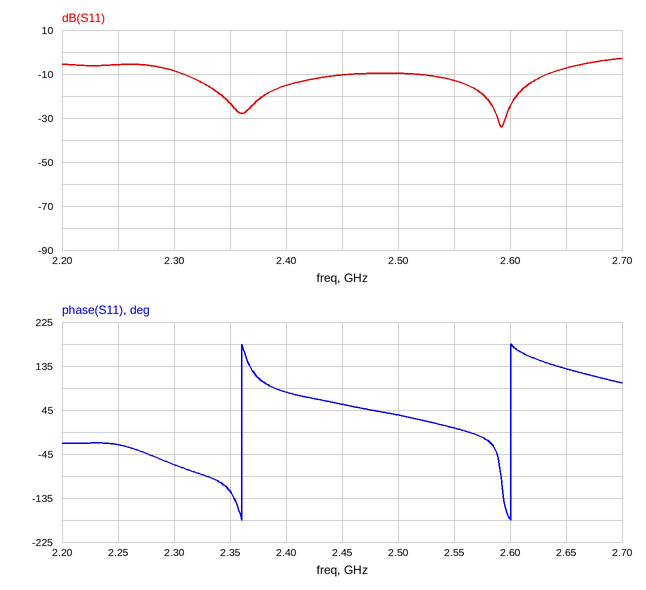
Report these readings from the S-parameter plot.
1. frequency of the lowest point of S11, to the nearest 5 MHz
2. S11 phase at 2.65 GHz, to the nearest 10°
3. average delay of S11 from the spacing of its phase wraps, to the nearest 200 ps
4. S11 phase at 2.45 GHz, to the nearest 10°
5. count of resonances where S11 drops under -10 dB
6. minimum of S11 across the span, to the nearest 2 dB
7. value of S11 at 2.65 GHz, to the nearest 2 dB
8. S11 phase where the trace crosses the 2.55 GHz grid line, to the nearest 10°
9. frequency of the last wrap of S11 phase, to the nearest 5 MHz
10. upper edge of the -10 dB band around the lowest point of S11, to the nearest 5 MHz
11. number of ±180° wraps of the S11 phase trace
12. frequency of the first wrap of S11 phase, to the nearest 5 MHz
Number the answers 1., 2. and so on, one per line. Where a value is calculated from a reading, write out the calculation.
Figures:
1. 2.590 GHz
2. 130°
3. 1 cycle / (2.600 GHz − 2.360 GHz) ≈ 4.2 ns
4. 60°
5. 2
6. -34 dB
7. -8 dB
8. 10°
9. 2.600 GHz
10. 2.635 GHz
11. 2
12. 2.360 GHz
